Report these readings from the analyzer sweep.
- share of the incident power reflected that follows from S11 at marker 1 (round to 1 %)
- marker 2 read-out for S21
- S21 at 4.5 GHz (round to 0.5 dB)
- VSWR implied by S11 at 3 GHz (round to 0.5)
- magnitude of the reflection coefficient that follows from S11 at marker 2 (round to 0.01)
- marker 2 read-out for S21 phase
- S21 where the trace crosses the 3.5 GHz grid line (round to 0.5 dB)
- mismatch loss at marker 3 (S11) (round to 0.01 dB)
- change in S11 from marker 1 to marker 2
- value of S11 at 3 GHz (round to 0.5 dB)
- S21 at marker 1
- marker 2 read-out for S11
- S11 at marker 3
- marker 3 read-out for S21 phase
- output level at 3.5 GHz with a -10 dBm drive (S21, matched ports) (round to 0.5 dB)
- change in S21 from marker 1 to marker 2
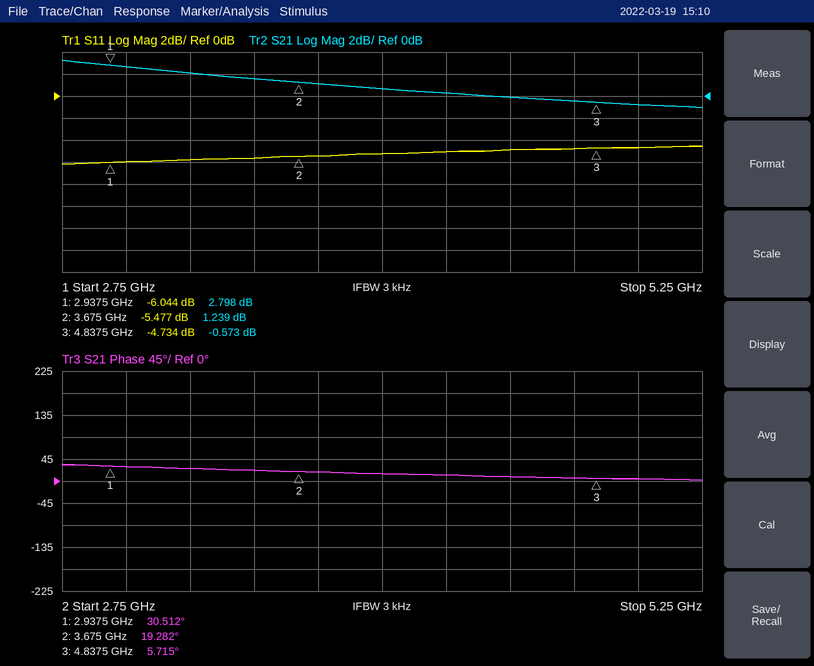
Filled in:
25 %
1.239 dB
0.0 dB
3.0
0.53
19.282°
1.5 dB
1.78 dB
0.567 dB
-6.0 dB
2.798 dB
-5.477 dB
-4.734 dB
5.715°
-8.5 dBm
-1.559 dB
